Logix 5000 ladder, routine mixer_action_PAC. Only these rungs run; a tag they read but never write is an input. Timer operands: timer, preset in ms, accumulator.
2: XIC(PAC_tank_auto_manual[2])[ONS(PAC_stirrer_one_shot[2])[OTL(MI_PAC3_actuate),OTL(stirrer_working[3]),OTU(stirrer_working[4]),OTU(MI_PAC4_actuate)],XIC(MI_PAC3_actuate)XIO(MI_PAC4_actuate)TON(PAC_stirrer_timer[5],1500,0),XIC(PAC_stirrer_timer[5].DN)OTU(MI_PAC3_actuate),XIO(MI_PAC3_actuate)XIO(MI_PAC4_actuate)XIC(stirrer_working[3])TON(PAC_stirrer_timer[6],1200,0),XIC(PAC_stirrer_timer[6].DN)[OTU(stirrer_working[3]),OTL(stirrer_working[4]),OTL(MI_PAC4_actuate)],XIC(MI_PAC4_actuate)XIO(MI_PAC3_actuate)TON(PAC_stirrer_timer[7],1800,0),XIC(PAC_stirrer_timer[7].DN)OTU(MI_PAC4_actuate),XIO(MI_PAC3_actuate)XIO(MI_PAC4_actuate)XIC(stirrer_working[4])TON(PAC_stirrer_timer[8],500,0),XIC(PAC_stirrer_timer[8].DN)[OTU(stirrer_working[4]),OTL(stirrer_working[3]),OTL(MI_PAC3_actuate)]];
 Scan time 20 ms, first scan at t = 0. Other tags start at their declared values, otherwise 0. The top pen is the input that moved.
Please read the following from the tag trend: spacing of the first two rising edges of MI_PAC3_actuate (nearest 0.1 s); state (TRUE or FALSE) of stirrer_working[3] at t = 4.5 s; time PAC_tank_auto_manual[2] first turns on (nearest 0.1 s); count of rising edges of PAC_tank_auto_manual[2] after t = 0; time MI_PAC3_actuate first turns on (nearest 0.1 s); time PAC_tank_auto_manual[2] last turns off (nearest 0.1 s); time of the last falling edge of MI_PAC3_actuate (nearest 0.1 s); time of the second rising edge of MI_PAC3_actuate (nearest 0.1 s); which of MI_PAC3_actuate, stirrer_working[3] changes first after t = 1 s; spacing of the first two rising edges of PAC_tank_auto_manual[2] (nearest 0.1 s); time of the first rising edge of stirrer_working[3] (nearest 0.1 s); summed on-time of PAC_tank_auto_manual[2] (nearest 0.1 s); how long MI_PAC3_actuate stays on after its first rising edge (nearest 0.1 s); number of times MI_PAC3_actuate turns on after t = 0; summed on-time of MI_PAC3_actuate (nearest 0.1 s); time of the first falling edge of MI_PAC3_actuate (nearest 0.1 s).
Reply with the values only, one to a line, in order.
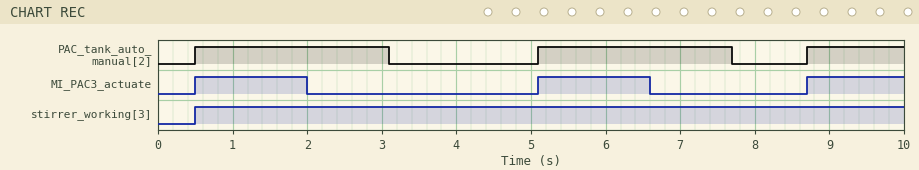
4.6 s
TRUE
0.5 s
3
0.5 s
7.7 s
6.6 s
5.1 s
MI_PAC3_actuate
4.6 s
0.5 s
6.5 s
1.5 s
3
4.3 s
2.0 s
